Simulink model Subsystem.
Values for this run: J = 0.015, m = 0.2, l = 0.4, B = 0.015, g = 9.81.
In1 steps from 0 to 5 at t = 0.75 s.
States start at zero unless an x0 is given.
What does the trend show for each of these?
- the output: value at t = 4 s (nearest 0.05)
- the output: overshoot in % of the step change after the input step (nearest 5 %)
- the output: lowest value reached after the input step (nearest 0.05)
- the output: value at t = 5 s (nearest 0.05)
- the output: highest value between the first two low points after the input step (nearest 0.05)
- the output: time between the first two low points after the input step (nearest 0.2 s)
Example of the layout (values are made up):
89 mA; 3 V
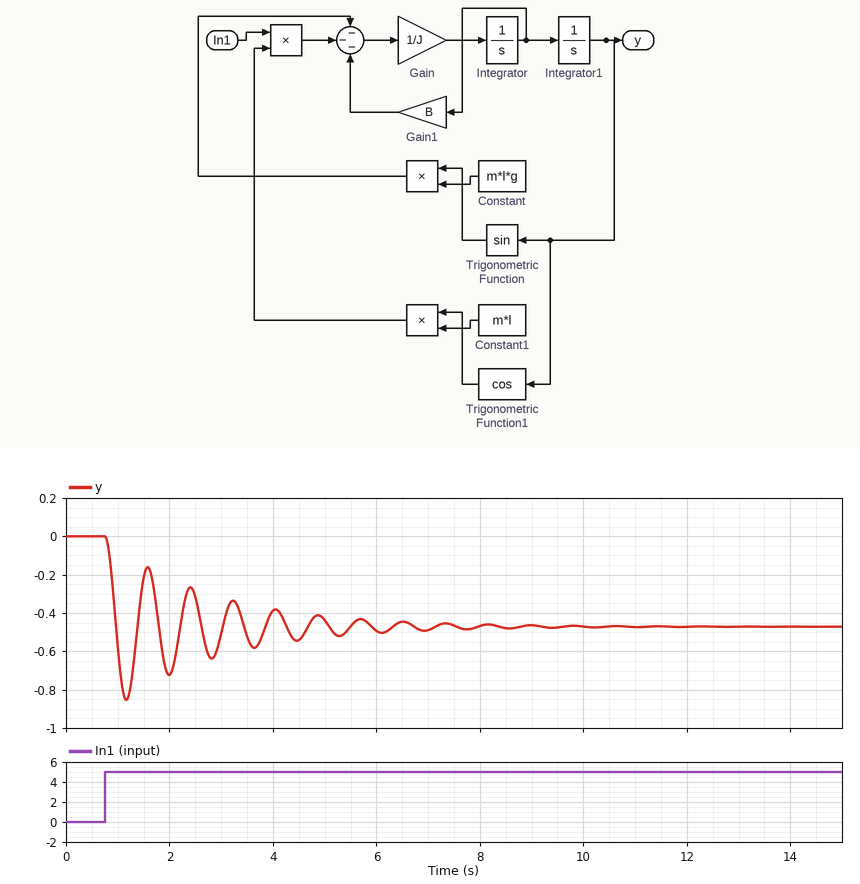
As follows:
-0.40; 80 %; -0.85; -0.45; -0.15; 0.8 s
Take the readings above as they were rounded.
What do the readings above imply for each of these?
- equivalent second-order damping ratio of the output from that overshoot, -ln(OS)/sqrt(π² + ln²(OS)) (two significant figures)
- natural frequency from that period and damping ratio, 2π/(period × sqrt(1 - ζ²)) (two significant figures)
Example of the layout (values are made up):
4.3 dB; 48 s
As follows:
0.071; 7.9 rad/s
